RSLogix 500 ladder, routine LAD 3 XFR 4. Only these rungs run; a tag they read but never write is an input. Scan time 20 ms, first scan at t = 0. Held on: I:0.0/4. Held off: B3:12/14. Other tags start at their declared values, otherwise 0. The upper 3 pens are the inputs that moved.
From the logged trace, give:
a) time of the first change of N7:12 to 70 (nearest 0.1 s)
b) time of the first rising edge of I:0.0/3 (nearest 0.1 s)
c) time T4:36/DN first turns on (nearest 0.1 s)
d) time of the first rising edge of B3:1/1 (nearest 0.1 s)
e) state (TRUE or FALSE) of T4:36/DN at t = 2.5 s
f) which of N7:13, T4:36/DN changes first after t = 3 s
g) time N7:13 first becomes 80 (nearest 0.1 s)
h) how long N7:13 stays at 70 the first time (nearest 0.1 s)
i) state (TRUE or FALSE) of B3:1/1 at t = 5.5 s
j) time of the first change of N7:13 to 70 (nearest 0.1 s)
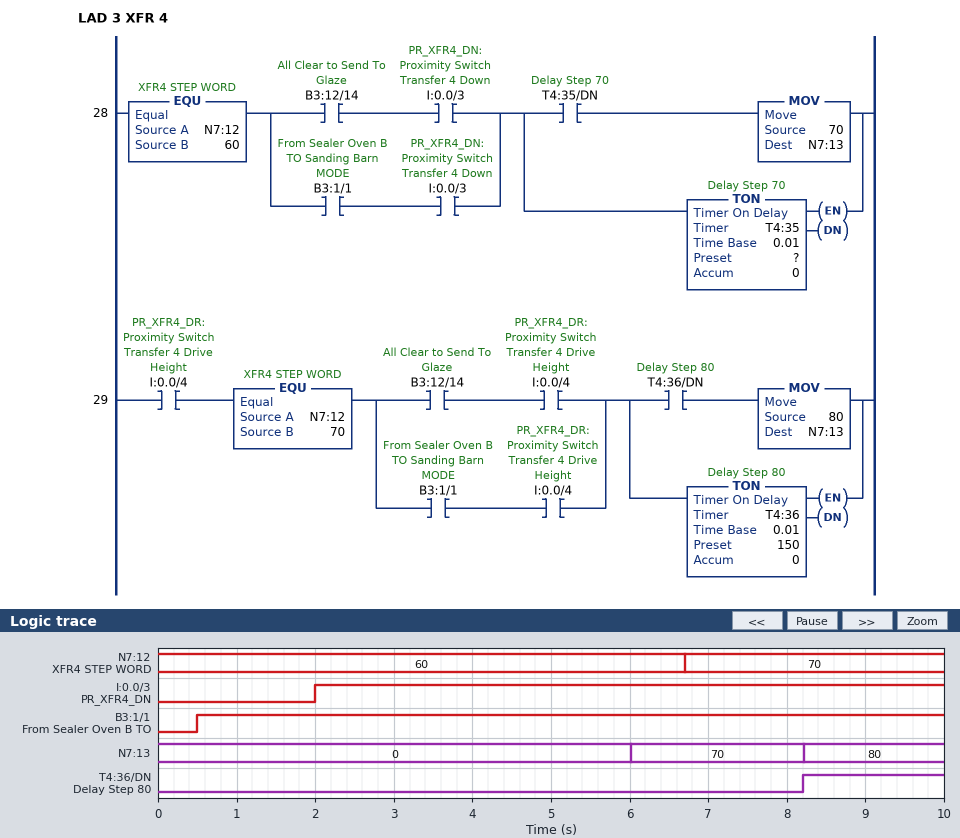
6.7 s
2.0 s
8.2 s
0.5 s
FALSE
N7:13
8.2 s
2.2 s
TRUE
6.0 s
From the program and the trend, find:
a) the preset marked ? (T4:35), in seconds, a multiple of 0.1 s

4.0 s
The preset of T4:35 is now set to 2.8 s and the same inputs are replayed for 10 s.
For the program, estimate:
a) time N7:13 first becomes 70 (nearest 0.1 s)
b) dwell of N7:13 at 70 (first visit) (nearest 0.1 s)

4.8 s
3.4 s
